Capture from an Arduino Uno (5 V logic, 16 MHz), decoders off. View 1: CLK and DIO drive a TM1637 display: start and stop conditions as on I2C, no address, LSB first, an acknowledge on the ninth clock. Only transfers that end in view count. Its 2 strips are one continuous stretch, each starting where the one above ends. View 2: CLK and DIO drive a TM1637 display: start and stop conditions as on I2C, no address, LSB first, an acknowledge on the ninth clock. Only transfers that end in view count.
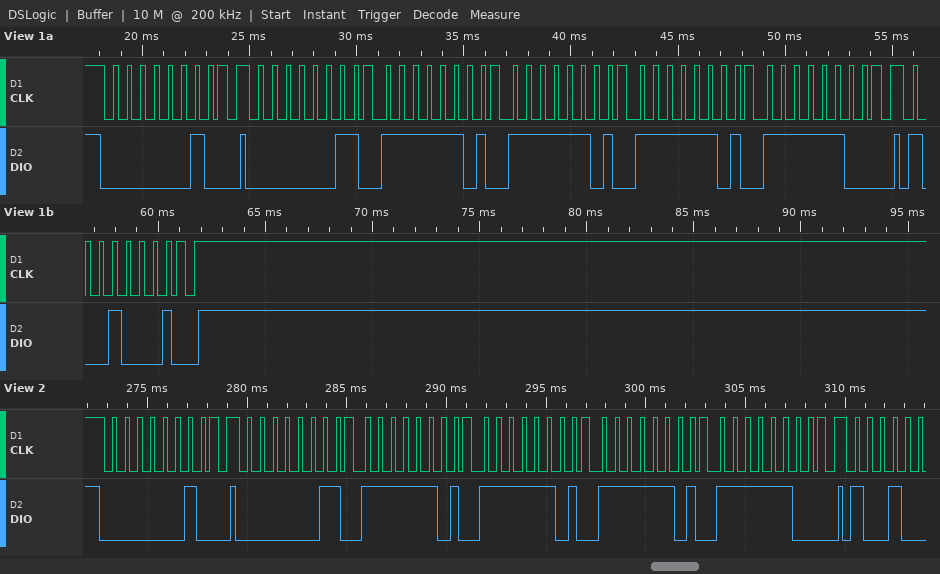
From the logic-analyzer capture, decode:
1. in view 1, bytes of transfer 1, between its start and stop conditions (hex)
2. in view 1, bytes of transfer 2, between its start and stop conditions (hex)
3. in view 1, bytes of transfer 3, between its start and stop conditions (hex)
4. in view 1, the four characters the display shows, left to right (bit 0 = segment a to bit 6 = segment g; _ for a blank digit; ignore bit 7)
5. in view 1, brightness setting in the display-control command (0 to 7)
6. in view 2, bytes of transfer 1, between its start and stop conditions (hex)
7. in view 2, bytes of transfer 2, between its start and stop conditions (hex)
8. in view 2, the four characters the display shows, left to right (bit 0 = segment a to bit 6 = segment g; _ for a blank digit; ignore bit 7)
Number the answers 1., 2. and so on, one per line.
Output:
1. 40
2. C0 BF BF BF 3F
3. 89
4. 0000
5. 1
6. 40
7. C0 BF BF BF 3F
8. 0000
